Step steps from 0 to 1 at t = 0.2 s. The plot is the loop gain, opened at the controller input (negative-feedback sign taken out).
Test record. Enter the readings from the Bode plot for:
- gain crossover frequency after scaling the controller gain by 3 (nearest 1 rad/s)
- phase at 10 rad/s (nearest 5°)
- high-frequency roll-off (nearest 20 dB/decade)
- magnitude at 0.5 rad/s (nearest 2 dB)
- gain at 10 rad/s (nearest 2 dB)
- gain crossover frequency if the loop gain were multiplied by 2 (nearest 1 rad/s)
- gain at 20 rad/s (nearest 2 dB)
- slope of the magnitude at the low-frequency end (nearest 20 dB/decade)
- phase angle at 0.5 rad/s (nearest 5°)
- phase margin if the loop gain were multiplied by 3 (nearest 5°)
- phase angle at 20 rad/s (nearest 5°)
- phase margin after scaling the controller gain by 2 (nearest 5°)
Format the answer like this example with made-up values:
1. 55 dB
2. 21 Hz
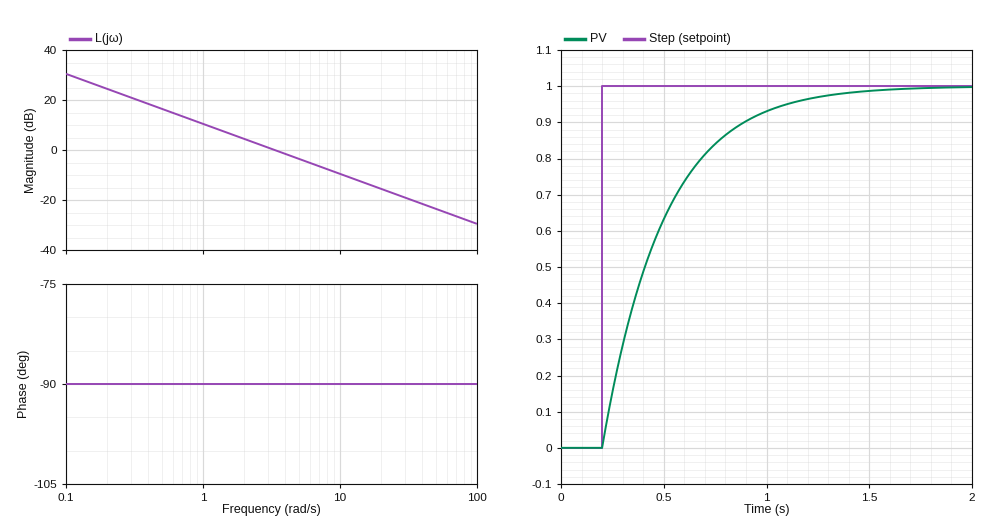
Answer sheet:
1. 10 rad/s
2. -90°
3. -20 dB/decade
4. 16 dB
5. -10 dB
6. 7 rad/s
7. -16 dB
8. -20 dB/decade
9. -90°
10. 90°
11. -90°
12. 90°
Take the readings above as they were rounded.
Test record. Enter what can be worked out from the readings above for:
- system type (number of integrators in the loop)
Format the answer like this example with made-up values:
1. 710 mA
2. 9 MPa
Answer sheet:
1. 1
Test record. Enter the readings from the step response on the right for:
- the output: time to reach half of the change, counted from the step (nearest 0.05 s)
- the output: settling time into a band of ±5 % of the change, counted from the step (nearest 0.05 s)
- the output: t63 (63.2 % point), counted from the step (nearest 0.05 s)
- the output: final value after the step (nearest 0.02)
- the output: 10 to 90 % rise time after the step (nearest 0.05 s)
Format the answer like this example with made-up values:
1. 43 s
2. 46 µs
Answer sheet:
1. 0.20 s
2. 0.90 s
3. 0.30 s
4. 1.00
5. 0.65 s
